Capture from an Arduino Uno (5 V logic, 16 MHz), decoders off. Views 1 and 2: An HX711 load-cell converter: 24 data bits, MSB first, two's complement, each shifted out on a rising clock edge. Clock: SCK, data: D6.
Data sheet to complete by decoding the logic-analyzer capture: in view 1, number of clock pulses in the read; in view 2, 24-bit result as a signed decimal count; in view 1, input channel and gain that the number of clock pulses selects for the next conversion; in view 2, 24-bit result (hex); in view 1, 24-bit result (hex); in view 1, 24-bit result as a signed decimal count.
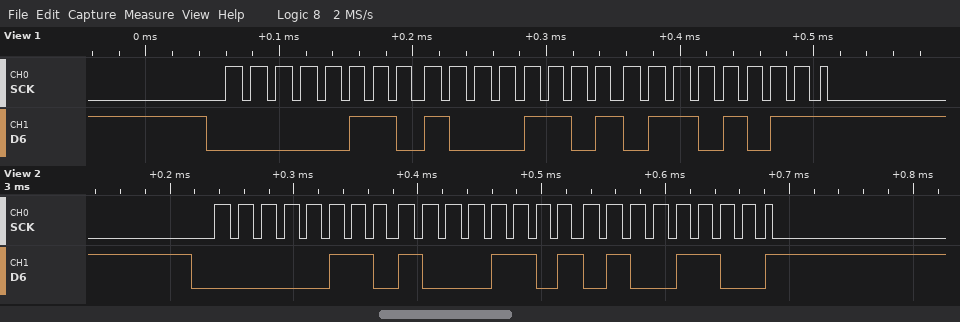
25
429388
channel A, gain 128
0x068D4C
0x068D6B
429419
